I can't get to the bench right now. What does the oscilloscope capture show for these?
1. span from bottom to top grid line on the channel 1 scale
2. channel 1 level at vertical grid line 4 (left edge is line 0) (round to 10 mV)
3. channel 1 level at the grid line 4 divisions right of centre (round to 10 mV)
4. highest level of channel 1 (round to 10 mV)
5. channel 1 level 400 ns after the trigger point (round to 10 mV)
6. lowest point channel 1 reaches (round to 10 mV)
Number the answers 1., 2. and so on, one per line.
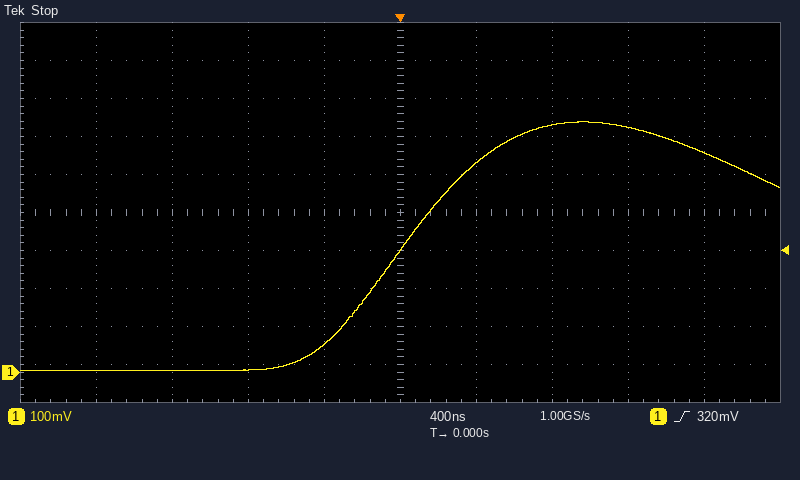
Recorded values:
1. 1 V
2. 70 mV
3. 580 mV
4. 660 mV
5. 550 mV
6. 0 mV
